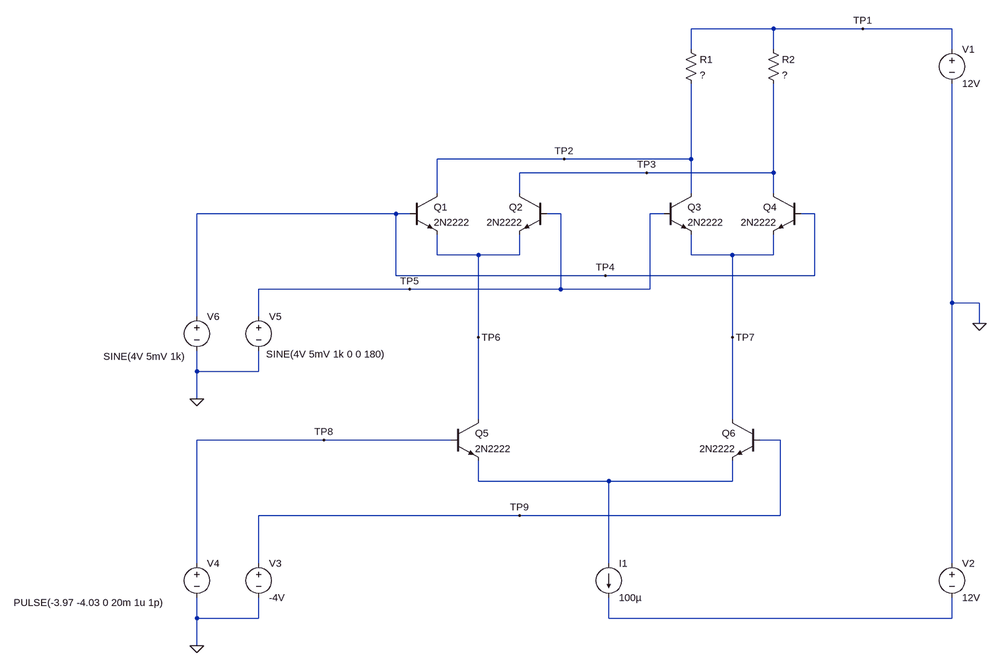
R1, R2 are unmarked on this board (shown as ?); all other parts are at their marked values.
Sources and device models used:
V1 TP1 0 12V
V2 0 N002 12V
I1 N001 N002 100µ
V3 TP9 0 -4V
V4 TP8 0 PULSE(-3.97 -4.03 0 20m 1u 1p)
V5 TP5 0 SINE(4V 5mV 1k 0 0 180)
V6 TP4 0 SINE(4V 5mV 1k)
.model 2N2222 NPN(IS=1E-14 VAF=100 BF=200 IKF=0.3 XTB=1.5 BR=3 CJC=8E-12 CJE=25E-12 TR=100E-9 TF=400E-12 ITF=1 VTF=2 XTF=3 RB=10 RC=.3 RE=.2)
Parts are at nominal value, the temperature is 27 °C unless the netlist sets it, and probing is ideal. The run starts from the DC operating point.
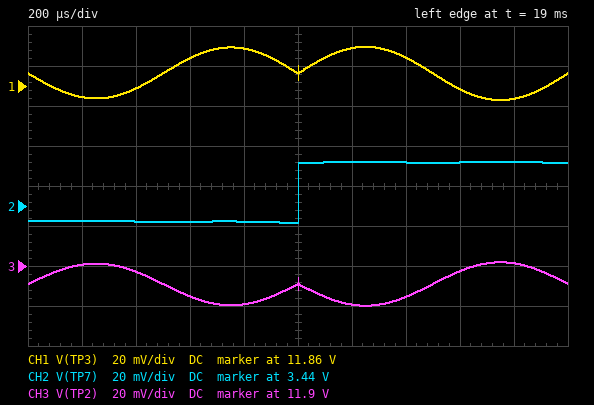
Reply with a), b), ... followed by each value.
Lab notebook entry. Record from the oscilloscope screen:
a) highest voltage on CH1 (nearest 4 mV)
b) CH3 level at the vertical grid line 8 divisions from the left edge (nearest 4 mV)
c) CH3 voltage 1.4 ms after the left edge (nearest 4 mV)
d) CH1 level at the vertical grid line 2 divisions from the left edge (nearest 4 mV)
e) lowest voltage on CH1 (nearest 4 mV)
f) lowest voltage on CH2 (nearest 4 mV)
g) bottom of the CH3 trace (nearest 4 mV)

a) 11.880 V
b) 11.896 V
c) 11.884 V
d) 11.860 V
e) 11.852 V
f) 3.432 V
g) 11.880 V
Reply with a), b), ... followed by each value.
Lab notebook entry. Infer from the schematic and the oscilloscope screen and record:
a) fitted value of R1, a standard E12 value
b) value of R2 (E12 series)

a) 2.2 kΩ
b) 2.7 kΩ
